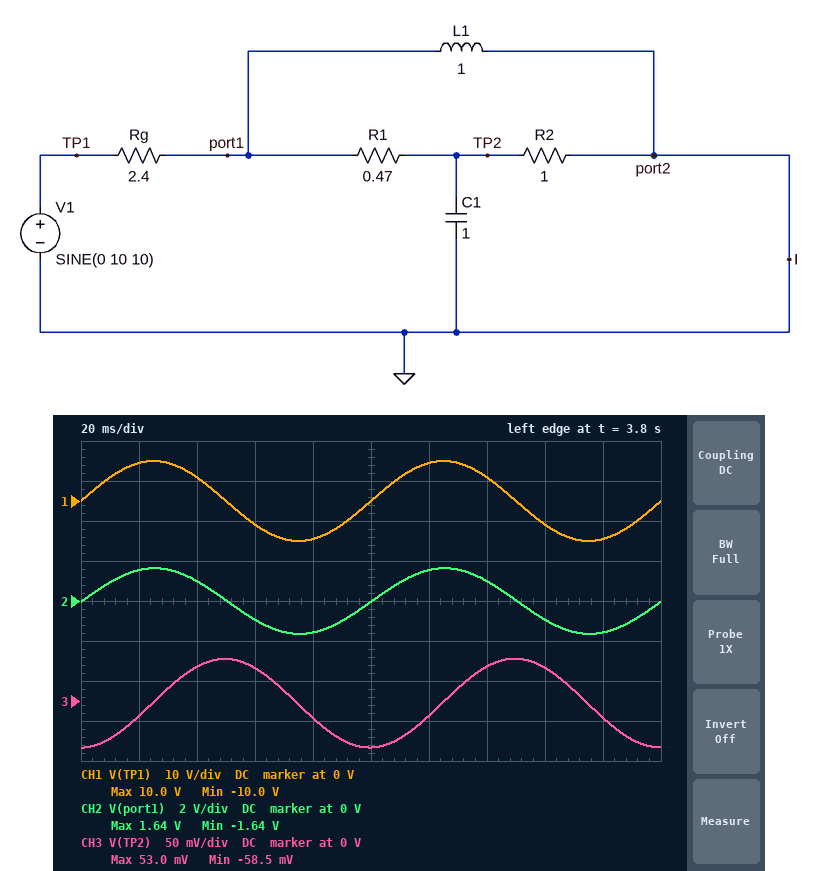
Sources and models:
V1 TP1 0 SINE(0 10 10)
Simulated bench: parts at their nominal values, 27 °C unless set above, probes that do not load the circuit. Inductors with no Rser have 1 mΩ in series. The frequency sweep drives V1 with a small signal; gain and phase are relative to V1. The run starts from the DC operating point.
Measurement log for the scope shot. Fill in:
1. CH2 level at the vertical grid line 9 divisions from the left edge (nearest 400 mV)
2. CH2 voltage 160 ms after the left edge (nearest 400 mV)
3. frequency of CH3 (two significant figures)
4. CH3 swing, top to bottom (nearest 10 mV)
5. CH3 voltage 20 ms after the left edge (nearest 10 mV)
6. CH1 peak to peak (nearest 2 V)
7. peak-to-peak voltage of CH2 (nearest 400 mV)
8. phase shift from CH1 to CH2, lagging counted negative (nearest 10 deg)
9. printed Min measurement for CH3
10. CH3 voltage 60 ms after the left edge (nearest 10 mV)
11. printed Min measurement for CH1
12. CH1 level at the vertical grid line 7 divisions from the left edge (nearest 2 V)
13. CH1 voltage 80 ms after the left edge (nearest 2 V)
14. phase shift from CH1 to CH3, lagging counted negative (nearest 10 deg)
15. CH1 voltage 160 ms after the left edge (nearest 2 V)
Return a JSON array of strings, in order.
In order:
["-1.6 V", "-800 mV", "10 Hz", "110 mV", "-20 mV", "20 V", "3.2 V", "0 deg", "-58.5 mV", "40 mV", "-10.0 V", "6 V", "-10 V", "-90 deg", "-6 V"]
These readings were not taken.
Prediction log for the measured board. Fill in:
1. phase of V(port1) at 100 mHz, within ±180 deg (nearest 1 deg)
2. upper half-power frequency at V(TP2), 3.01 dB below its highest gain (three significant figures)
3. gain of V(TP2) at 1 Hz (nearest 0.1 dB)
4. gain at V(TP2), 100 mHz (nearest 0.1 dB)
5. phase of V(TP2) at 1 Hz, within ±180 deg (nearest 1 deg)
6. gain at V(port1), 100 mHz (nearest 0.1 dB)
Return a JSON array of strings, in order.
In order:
["49 deg", "363 mHz", "-25.2 dB", "-16.0 dB", "-74 deg", "-12.5 dB"]
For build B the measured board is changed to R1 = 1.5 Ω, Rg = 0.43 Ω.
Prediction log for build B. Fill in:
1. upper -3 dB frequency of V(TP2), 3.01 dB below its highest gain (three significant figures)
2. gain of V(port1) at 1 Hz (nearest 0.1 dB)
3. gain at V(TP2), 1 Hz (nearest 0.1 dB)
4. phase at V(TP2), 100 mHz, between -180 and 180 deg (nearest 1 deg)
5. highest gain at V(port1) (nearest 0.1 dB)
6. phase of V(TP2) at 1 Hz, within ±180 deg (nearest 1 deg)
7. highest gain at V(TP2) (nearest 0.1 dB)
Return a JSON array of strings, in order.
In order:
["337 mHz", "-2.1 dB", "-21.9 dB", "8 deg", "-1.9 dB", "-73 deg", "-11.1 dB"]
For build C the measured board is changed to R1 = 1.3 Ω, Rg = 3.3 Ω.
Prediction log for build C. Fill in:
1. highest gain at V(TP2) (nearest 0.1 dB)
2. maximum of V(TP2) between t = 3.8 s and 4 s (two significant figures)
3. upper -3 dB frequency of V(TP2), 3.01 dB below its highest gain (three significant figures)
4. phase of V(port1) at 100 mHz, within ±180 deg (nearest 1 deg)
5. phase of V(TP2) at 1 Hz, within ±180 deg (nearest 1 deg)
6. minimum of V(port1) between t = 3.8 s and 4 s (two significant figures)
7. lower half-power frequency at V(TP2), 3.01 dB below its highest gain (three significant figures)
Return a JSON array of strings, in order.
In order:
["-19.9 dB", "34 mV", "438 mHz", "62 deg", "-70 deg", "-2.8 V", "95.5 mHz"]
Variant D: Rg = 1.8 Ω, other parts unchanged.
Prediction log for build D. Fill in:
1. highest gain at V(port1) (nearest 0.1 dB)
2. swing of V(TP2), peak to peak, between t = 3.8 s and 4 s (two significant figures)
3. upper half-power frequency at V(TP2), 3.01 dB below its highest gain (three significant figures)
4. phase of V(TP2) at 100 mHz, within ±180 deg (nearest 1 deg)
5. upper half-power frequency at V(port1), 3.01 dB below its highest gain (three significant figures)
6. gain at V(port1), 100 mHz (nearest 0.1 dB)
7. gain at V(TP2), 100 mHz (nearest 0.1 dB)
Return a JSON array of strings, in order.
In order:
["-8.4 dB", "140 mV", "369 mHz", "34 deg", "546 mHz", "-10.4 dB", "-13.9 dB"]
